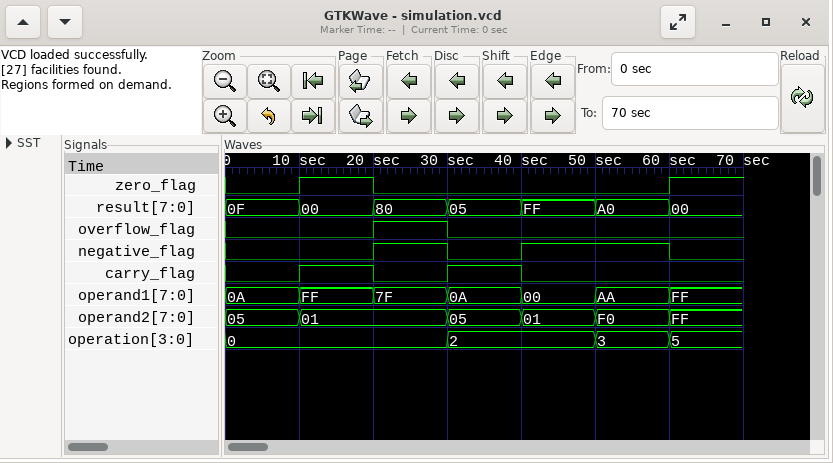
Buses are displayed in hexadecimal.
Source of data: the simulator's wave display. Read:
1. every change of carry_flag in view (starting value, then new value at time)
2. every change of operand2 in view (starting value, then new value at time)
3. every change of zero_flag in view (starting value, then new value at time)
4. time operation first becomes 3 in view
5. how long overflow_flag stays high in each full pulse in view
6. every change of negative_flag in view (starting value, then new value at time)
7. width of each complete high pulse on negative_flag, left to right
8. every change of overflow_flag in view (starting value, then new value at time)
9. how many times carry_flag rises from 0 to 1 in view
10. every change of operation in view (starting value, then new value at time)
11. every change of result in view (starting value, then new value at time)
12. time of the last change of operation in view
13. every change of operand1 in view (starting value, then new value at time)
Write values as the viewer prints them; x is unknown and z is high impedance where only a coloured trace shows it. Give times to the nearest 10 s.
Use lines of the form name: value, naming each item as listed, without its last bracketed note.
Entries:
every change of carry_flag in view: 0, 1 at 10 s, 0 at 20 s, 1 at 30 s, 0 at 40 s
every change of operand2 in view: 05, 01 at 10 s, 05 at 30 s, 01 at 40 s, F0 at 50 s, FF at 60 s
every change of zero_flag in view: 0, 1 at 10 s, 0 at 20 s, 1 at 60 s
time operation first becomes 3 in view: 50 s
how long overflow_flag stays high in each full pulse in view: 10 s
every change of negative_flag in view: 0, 1 at 20 s, 0 at 30 s, 1 at 40 s, 0 at 60 s
width of each complete high pulse on negative_flag, left to right: 10 s, 20 s
every change of overflow_flag in view: 0, 1 at 20 s, 0 at 30 s
how many times carry_flag rises from 0 to 1 in view: 2
every change of operation in view: 0, 2 at 30 s, 3 at 50 s, 5 at 60 s
every change of result in view: 0F, 00 at 10 s, 80 at 20 s, 05 at 30 s, FF at 40 s, A0 at 50 s, 00 at 60 s
time of the last change of operation in view: 60 s
every change of operand1 in view: 0A, FF at 10 s, 7F at 20 s, 0A at 30 s, 00 at 40 s, AA at 50 s, FF at 60 s
